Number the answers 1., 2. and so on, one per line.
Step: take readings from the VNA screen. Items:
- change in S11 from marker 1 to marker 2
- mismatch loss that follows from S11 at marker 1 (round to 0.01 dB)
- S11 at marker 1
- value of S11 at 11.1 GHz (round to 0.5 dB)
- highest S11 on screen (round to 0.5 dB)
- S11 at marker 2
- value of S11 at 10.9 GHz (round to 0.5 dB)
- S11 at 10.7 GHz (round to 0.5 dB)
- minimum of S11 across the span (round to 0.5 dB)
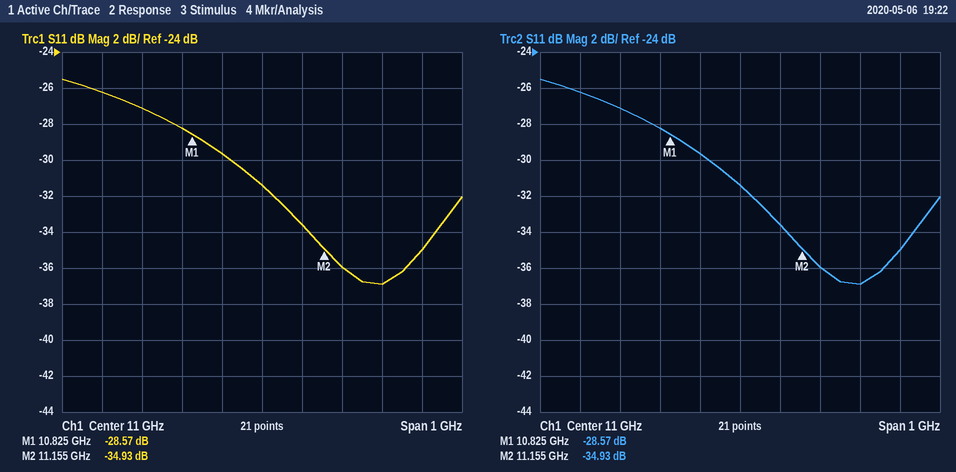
1. -6.36 dB
2. 0.01 dB
3. -28.57 dB
4. -33.5 dB
5. -25.5 dB
6. -34.93 dB
7. -29.5 dB
8. -27.0 dB
9. -37.0 dB
